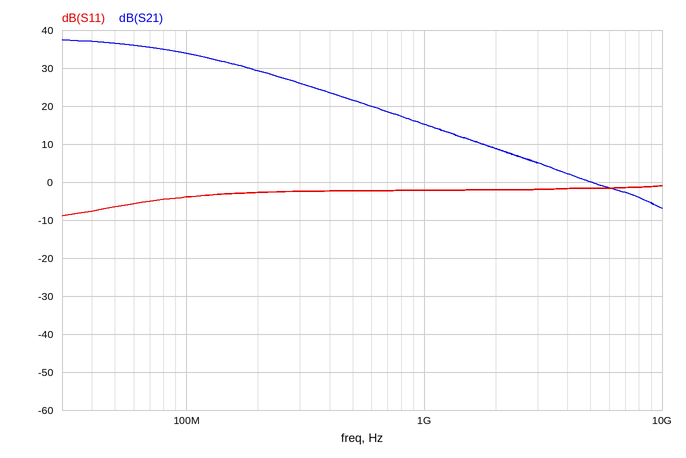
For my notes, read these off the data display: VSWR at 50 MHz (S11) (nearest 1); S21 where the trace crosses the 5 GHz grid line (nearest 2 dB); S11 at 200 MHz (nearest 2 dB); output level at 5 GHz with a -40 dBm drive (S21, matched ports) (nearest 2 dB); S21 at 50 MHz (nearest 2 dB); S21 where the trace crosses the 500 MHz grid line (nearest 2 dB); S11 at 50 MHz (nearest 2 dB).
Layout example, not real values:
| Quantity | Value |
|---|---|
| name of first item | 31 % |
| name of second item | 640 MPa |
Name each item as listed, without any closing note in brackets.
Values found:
| Quantity | Value |
|---|---|
| VSWR at 50 MHz (S11) | 3 |
| S21 where the trace crosses the 5 GHz grid line | 0 dB |
| S11 at 200 MHz | -2 dB |
| output level at 5 GHz with a -40 dBm drive (S21, matched ports) | -40 dBm |
| S21 at 50 MHz | 36 dB |
| S21 where the trace crosses the 500 MHz grid line | 22 dB |
| S11 at 50 MHz | -6 dB |
